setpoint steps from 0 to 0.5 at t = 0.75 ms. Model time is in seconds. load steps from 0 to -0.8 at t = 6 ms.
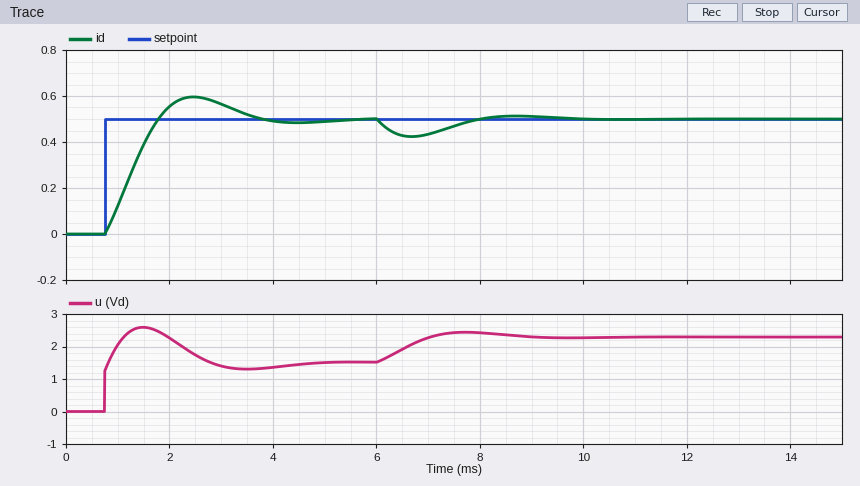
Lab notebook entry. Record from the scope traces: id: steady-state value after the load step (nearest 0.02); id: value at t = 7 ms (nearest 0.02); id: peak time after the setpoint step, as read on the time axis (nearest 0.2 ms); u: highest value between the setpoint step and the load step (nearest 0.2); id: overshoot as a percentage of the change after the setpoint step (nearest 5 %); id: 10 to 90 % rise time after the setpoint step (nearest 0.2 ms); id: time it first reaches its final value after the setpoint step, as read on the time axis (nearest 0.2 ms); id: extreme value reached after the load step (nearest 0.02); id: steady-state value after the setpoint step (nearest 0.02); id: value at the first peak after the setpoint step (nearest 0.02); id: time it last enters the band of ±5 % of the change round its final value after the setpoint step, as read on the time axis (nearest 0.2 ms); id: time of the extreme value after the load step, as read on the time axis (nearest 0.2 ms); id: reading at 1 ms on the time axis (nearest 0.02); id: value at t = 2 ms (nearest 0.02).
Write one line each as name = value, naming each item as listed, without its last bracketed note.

id: steady-state value after the load step = 0.50
id: value at t = 7 ms = 0.44
id: peak time after the setpoint step, as read on the time axis = 2.4 ms
u: highest value between the setpoint step and the load step = 2.6
id: overshoot as a percentage of the change after the setpoint step = 20 %
id: 10 to 90 % rise time after the setpoint step = 0.8 ms
id: time it first reaches its final value after the setpoint step, as read on the time axis = 1.8 ms
id: extreme value reached after the load step = 0.42
id: steady-state value after the setpoint step = 0.50
id: value at the first peak after the setpoint step = 0.60
id: time it last enters the band of ±5 % of the change round its final value after the setpoint step, as read on the time axis = 3.4 ms
id: time of the extreme value after the load step, as read on the time axis = 6.6 ms
id: reading at 1 ms on the time axis = 0.12
id: value at t = 2 ms = 0.56
